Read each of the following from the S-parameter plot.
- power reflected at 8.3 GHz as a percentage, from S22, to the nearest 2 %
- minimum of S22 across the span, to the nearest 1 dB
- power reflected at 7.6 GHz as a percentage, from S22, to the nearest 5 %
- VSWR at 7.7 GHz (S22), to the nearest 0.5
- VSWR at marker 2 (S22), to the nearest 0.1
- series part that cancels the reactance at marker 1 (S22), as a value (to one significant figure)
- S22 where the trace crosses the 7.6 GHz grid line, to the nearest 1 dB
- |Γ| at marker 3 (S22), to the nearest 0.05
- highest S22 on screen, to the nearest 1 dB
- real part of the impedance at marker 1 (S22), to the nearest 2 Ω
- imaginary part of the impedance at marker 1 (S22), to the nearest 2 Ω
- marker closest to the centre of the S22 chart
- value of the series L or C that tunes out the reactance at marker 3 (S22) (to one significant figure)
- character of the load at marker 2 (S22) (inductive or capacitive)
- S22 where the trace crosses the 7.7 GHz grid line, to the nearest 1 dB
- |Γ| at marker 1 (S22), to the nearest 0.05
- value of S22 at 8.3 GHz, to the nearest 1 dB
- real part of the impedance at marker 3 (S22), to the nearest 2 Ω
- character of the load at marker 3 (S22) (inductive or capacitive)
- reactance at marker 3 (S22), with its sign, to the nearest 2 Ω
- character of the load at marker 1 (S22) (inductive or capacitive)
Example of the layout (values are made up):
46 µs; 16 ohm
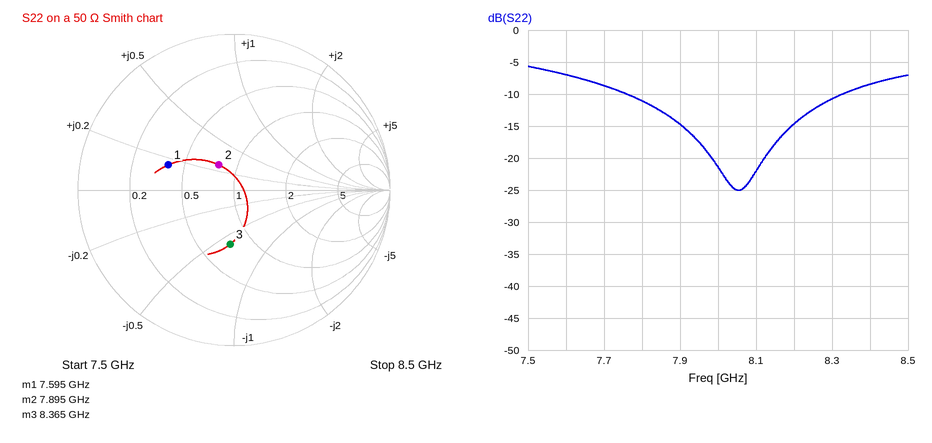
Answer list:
8 %; -25 dB; 20 %; 2.0; 1.5; 3 pF; -7 dB; 0.35; -6 dB; 20 Ω; +8 Ω; marker 2; 600 pH; inductive; -9 dB; 0.45; -11 dB; 38 Ω; capacitive; -30 Ω; inductive
